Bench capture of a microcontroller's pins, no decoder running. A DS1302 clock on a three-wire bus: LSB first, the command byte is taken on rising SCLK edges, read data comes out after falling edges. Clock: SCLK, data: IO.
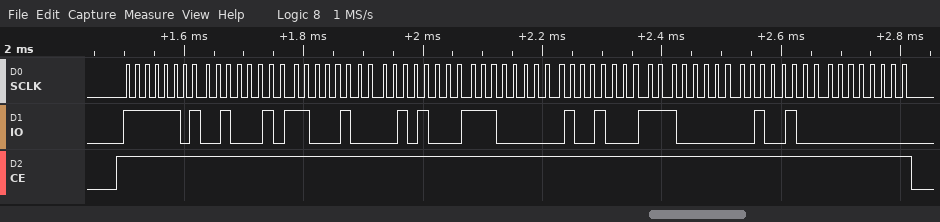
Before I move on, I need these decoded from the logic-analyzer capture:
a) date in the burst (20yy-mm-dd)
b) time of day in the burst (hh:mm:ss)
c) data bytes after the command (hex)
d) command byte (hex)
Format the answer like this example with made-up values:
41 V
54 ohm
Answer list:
2024-12-07
14:23:44
44 23 14 07 12 07 24 00
0xBF
